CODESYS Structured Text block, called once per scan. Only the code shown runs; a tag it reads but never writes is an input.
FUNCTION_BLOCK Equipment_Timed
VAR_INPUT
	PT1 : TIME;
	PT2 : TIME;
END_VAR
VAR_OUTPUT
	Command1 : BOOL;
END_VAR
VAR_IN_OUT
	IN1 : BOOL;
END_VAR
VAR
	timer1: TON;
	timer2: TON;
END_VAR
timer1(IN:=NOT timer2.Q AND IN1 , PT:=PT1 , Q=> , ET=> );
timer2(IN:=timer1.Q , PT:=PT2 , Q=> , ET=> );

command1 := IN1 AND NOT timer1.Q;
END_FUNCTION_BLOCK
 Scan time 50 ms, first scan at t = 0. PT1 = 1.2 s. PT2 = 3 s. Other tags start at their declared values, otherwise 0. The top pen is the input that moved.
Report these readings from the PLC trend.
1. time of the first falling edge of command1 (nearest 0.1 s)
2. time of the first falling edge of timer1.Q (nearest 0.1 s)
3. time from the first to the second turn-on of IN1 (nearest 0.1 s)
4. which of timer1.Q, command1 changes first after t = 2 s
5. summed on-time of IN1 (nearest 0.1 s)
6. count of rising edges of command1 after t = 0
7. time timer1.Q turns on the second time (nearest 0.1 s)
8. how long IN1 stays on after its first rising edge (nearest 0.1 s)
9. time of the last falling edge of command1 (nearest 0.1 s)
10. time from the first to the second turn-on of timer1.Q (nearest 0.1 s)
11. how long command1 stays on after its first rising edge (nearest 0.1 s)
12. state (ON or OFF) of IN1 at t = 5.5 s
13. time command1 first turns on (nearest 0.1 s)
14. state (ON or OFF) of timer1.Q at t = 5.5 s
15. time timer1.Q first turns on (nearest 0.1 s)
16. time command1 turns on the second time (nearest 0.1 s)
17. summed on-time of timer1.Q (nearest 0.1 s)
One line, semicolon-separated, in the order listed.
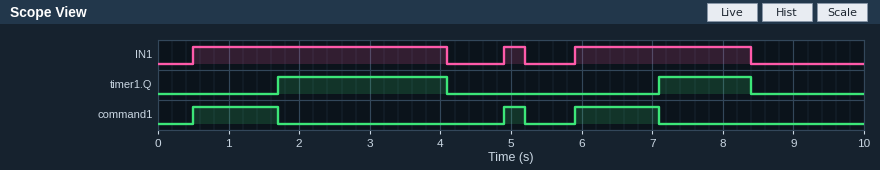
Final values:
1.7 s; 4.1 s; 4.4 s; timer1.Q; 6.4 s; 3; 7.1 s; 3.6 s; 7.1 s; 5.4 s; 1.2 s; OFF; 0.5 s; OFF; 1.7 s; 4.9 s; 3.7 s
